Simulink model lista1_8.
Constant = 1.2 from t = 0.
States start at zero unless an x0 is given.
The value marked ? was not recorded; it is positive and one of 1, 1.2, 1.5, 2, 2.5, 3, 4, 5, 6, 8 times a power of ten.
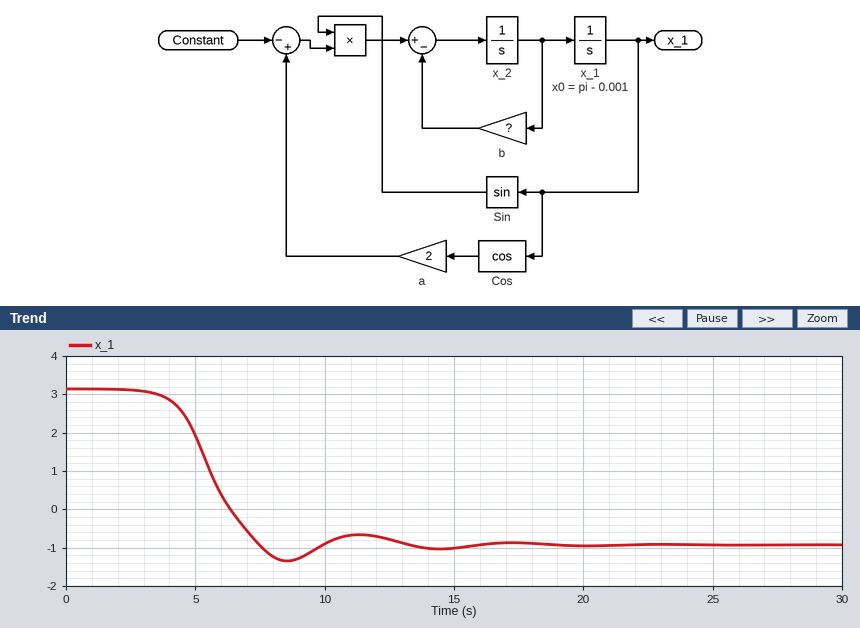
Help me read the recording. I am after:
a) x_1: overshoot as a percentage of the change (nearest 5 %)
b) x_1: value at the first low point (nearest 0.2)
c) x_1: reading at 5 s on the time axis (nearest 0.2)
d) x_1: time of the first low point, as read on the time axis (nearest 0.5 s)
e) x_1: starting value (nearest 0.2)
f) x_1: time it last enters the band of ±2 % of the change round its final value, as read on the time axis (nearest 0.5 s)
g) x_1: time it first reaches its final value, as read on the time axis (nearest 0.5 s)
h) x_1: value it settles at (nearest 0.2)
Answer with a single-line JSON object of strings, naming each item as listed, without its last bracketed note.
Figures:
{"x_1: overshoot as a percentage of the change": "10 %", "x_1: value at the first low point": "-1.4", "x_1: reading at 5 s on the time axis": "2.0", "x_1: time of the first low point, as read on the time axis": "8.5 s", "x_1: starting value": "3.2", "x_1: time it last enters the band of ±2 % of the change round its final value, as read on the time axis": "15.0 s", "x_1: time it first reaches its final value, as read on the time axis": "7.5 s", "x_1: value it settles at": "-1.0"}
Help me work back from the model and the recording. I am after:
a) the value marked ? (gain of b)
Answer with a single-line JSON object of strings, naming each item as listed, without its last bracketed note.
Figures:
{"the value marked ?": "0.5"}
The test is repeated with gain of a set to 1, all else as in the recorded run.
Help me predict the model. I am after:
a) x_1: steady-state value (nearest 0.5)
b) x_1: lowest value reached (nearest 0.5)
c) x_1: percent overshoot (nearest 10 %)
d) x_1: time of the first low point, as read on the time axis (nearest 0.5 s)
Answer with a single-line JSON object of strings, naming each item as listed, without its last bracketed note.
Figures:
{"x_1: steady-state value": "0.0", "x_1: lowest value reached": "-1.0", "x_1: percent overshoot": "30 %", "x_1: time of the first low point, as read on the time axis": "9.5 s"}
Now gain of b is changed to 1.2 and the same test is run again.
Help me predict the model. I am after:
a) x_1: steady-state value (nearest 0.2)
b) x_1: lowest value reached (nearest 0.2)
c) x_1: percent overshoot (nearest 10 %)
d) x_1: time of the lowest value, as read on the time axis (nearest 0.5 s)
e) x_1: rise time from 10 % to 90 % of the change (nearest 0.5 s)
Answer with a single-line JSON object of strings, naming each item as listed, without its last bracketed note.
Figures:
{"x_1: steady-state value": "1.0", "x_1: lowest value reached": "0.6", "x_1: percent overshoot": "20 %", "x_1: time of the lowest value, as read on the time axis": "8.0 s", "x_1: rise time from 10 % to 90 % of the change": "2.0 s"}
